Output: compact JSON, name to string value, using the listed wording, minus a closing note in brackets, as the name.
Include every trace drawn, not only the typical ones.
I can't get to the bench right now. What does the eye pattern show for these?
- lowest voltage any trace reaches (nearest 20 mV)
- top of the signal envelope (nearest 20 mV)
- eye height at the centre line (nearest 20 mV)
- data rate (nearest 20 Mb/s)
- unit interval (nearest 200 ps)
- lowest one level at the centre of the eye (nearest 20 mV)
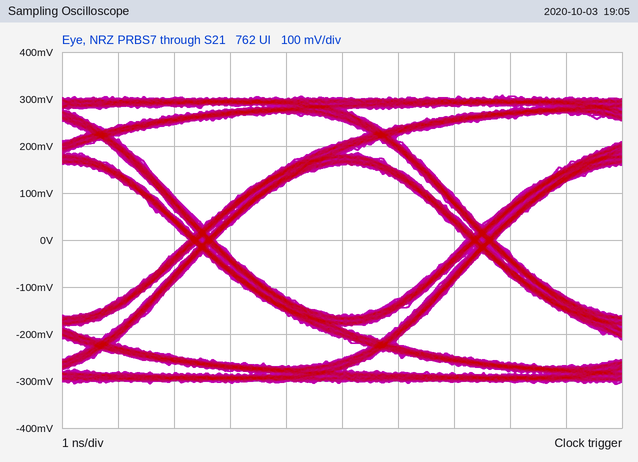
{"lowest voltage any trace reaches": "-300 mV", "top of the signal envelope": "300 mV", "eye height at the centre line": "320 mV", "data rate": "200 Mb/s", "unit interval": "5.0 ns", "lowest one level at the centre of the eye": "160 mV"}
